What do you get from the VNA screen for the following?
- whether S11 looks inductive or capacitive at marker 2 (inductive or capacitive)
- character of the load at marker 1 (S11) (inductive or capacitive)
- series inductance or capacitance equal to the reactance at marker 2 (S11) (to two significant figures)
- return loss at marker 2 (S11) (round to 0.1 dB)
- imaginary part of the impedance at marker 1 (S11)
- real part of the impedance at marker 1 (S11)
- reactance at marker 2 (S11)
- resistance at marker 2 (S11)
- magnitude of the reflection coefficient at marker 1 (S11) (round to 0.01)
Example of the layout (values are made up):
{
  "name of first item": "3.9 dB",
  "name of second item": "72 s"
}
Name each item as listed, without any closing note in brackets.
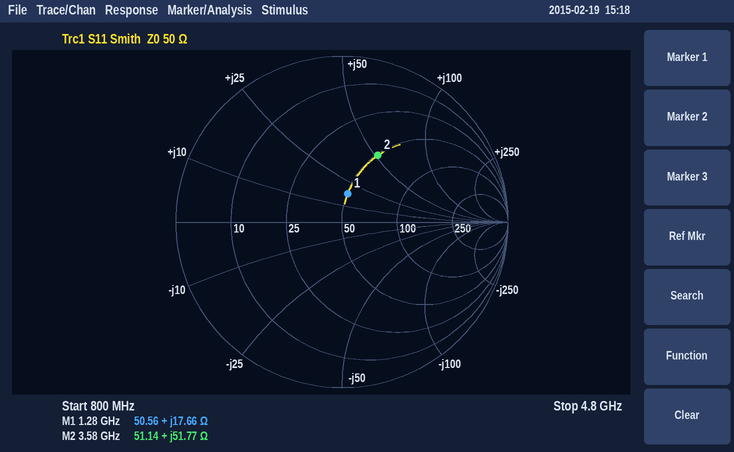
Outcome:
{
  "whether S11 looks inductive or capacitive at marker 2": "inductive",
  "character of the load at marker 1 (S11)": "inductive",
  "series inductance or capacitance equal to the reactance at marker 2 (S11)": "2.3 nH",
  "return loss at marker 2 (S11)": "6.8 dB",
  "imaginary part of the impedance at marker 1": "+17.66 Ω",
  "real part of the impedance at marker 1": "50.56 Ω",
  "reactance at marker 2": "+51.77 Ω",
  "resistance at marker 2": "51.14 Ω",
  "magnitude of the reflection coefficient at marker 1 (S11)": "0.17"
}
